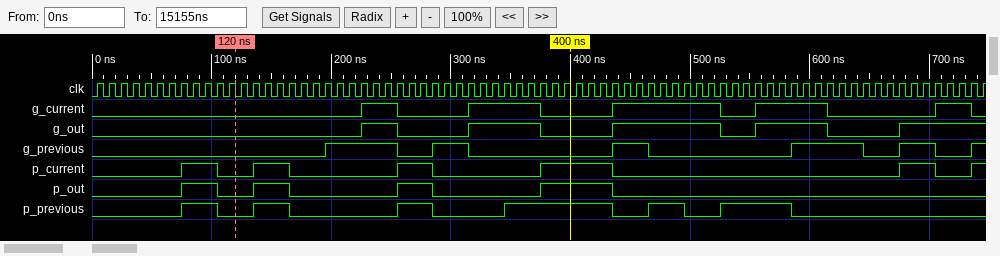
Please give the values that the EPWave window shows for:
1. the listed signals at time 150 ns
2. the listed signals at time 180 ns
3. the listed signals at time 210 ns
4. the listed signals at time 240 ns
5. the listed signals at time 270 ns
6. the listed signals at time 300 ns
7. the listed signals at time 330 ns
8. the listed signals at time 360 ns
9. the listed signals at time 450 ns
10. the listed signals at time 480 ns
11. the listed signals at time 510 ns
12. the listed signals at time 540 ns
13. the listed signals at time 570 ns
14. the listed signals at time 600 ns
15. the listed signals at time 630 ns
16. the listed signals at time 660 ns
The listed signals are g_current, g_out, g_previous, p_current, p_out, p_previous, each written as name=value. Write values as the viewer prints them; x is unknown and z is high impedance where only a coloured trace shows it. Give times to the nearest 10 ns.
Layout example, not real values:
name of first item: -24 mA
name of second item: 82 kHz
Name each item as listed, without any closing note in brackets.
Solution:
the listed signals at time 150 ns: g_current=0, g_out=0, g_previous=0, p_current=1, p_out=1, p_previous=1
the listed signals at time 180 ns: g_current=0, g_out=0, g_previous=0, p_current=0, p_out=0, p_previous=0
the listed signals at time 210 ns: g_current=0, g_out=0, g_previous=1, p_current=0, p_out=0, p_previous=0
the listed signals at time 240 ns: g_current=1, g_out=1, g_previous=1, p_current=0, p_out=0, p_previous=0
the listed signals at time 270 ns: g_current=0, g_out=0, g_previous=0, p_current=1, p_out=1, p_previous=1
the listed signals at time 300 ns: g_current=0, g_out=0, g_previous=1, p_current=0, p_out=0, p_previous=0
the listed signals at time 330 ns: g_current=1, g_out=1, g_previous=0, p_current=0, p_out=0, p_previous=0
the listed signals at time 360 ns: g_current=1, g_out=1, g_previous=0, p_current=0, p_out=0, p_previous=1
the listed signals at time 450 ns: g_current=1, g_out=1, g_previous=1, p_current=0, p_out=0, p_previous=0
the listed signals at time 480 ns: g_current=1, g_out=1, g_previous=0, p_current=0, p_out=0, p_previous=1
the listed signals at time 510 ns: g_current=1, g_out=1, g_previous=0, p_current=0, p_out=0, p_previous=0
the listed signals at time 540 ns: g_current=0, g_out=0, g_previous=0, p_current=0, p_out=0, p_previous=1
the listed signals at time 570 ns: g_current=1, g_out=1, g_previous=0, p_current=0, p_out=0, p_previous=1
the listed signals at time 600 ns: g_current=1, g_out=1, g_previous=1, p_current=0, p_out=0, p_previous=0
the listed signals at time 630 ns: g_current=0, g_out=0, g_previous=1, p_current=0, p_out=0, p_previous=0
the listed signals at time 660 ns: g_current=0, g_out=0, g_previous=0, p_current=0, p_out=0, p_previous=0
